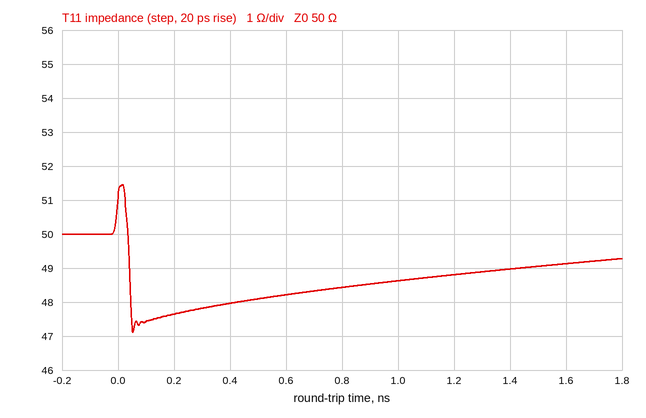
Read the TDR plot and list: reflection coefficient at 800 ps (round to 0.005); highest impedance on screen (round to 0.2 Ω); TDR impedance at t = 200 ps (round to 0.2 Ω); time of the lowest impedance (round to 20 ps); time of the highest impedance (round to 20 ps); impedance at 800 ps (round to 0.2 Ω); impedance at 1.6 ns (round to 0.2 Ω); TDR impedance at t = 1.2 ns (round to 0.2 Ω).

-0.015
51.4 Ω
47.6 Ω
60 ps
20 ps
48.4 Ω
49.2 Ω
48.8 Ω
